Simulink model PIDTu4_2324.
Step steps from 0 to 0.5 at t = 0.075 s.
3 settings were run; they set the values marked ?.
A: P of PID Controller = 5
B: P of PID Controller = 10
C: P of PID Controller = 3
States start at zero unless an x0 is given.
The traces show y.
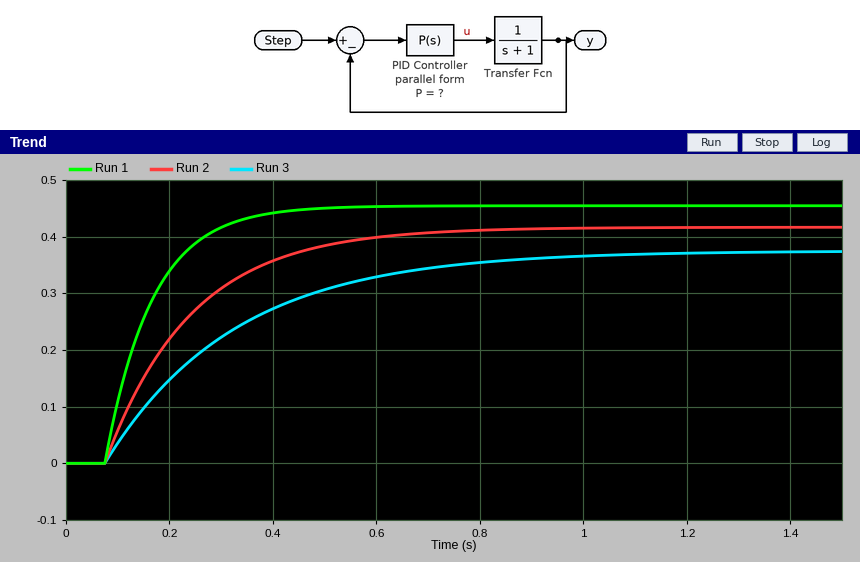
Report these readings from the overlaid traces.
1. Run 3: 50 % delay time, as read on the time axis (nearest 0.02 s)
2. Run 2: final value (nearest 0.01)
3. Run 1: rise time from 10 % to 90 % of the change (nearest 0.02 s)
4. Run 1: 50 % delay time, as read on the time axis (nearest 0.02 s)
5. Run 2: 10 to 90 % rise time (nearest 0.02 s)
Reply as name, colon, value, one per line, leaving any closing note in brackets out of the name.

Run 3: 50 % delay time, as read on the time axis: 0.24 s
Run 2: final value: 0.42
Run 1: rise time from 10 % to 90 % of the change: 0.20 s
Run 1: 50 % delay time, as read on the time axis: 0.14 s
Run 2: 10 to 90 % rise time: 0.36 s
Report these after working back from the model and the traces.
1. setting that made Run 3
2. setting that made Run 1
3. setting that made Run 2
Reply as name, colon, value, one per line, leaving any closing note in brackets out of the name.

setting that made Run 3: C
setting that made Run 1: B
setting that made Run 2: A
